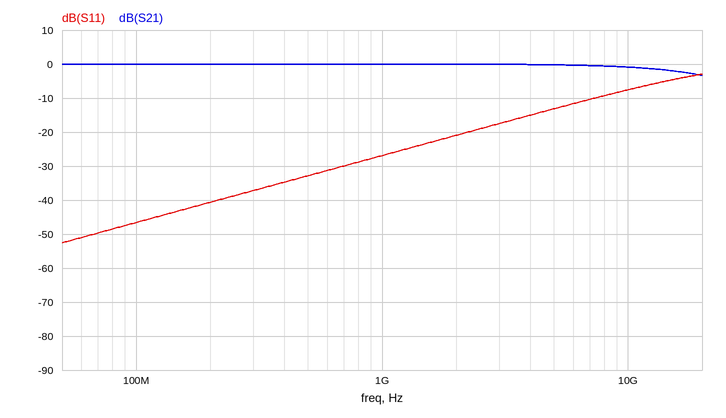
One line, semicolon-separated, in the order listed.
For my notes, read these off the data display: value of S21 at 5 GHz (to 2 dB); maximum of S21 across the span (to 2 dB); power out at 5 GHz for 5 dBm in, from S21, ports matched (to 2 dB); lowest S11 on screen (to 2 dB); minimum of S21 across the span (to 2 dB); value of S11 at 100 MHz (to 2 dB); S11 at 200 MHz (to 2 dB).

0 dB; 0 dB; 4 dBm; -52 dB; -4 dB; -46 dB; -40 dB
